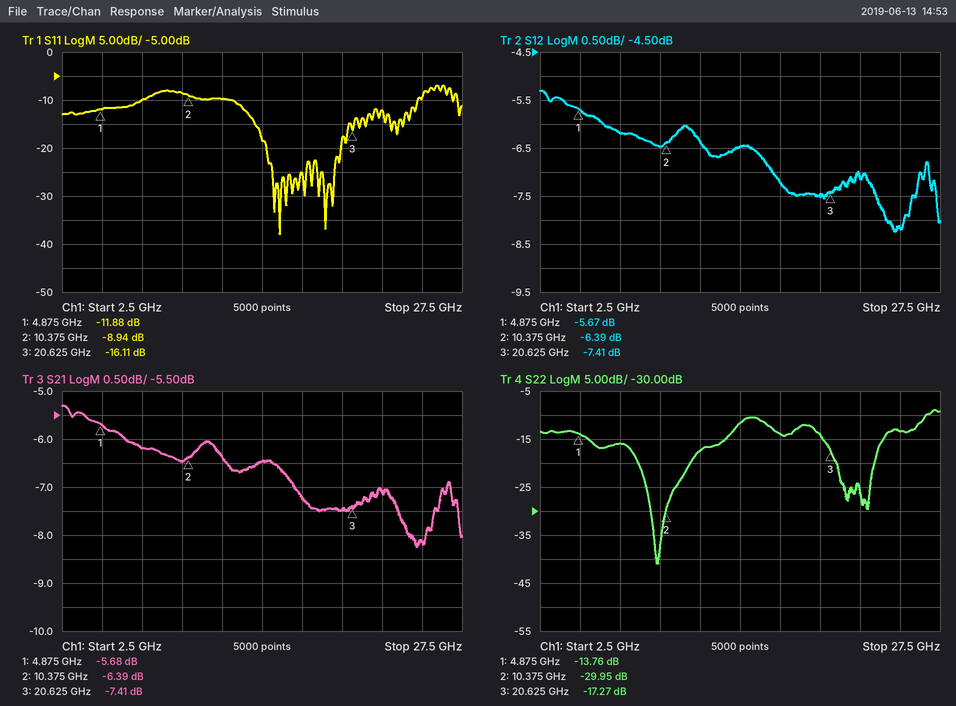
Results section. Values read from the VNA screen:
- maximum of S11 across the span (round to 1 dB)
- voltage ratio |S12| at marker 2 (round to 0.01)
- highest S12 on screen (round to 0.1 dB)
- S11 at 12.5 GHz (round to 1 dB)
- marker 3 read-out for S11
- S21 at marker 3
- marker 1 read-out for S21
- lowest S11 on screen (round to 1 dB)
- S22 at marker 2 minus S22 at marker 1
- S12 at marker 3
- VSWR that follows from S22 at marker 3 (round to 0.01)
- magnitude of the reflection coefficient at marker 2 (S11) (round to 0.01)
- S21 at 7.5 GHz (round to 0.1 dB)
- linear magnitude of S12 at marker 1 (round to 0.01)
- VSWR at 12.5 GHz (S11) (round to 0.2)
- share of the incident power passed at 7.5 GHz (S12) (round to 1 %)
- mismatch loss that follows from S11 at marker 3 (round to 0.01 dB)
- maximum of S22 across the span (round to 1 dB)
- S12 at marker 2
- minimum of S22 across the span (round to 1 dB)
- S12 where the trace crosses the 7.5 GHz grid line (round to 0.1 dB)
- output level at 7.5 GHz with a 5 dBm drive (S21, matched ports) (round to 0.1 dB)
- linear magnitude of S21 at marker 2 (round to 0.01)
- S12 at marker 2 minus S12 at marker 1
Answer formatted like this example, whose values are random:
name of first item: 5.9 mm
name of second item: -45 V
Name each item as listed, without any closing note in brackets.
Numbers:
maximum of S11 across the span: -7 dB
voltage ratio |S12| at marker 2: 0.48
highest S12 on screen: -5.3 dB
S11 at 12.5 GHz: -10 dB
marker 3 read-out for S11: -16.11 dB
S21 at marker 3: -7.41 dB
marker 1 read-out for S21: -5.68 dB
lowest S11 on screen: -38 dB
S22 at marker 2 minus S22 at marker 1: -16.19 dB
S12 at marker 3: -7.41 dB
VSWR that follows from S22 at marker 3: 1.32
magnitude of the reflection coefficient at marker 2 (S11): 0.36
S21 at 7.5 GHz: -6.2 dB
linear magnitude of S12 at marker 1: 0.52
VSWR at 12.5 GHz (S11): 2.0
share of the incident power passed at 7.5 GHz (S12): 24 %
mismatch loss that follows from S11 at marker 3: 0.11 dB
maximum of S22 across the span: -9 dB
S12 at marker 2: -6.39 dB
minimum of S22 across the span: -41 dB
S12 where the trace crosses the 7.5 GHz grid line: -6.2 dB
output level at 7.5 GHz with a 5 dBm drive (S21, matched ports): -1.2 dBm
linear magnitude of S21 at marker 2: 0.48
S12 at marker 2 minus S12 at marker 1: -0.72 dB
